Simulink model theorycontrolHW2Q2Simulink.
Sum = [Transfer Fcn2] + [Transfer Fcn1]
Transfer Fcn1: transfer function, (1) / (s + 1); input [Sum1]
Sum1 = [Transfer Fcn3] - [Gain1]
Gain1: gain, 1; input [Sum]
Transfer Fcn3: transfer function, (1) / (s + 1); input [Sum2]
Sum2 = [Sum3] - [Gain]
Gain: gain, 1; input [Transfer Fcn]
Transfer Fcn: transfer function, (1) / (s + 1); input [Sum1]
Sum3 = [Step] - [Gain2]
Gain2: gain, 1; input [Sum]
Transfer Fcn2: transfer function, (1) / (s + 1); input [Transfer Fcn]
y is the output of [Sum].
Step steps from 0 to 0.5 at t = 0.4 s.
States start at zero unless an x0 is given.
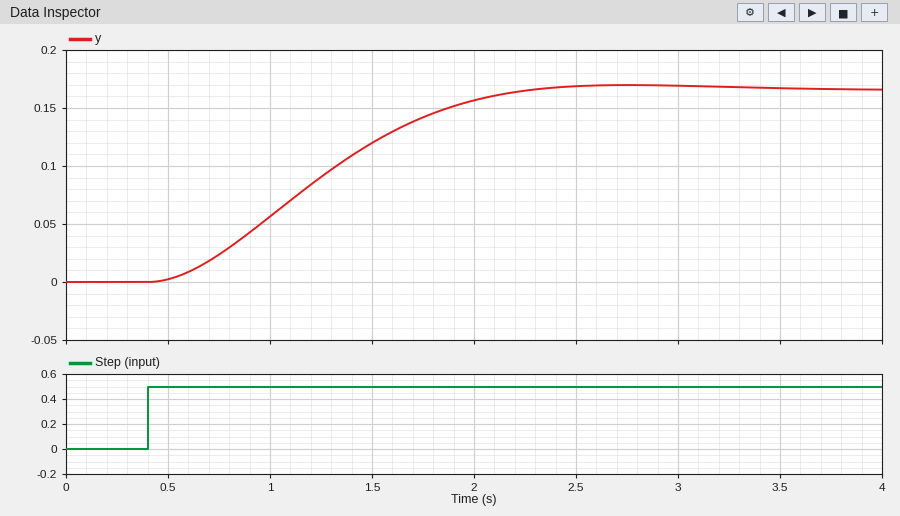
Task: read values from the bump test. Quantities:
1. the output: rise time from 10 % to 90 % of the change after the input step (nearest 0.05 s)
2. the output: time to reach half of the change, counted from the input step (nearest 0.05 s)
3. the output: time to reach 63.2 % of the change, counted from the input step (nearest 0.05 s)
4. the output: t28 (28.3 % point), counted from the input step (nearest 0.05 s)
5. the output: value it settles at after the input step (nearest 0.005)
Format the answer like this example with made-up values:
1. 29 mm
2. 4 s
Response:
1. 1.20 s
2. 0.80 s
3. 0.95 s
4. 0.55 s
5. 0.165
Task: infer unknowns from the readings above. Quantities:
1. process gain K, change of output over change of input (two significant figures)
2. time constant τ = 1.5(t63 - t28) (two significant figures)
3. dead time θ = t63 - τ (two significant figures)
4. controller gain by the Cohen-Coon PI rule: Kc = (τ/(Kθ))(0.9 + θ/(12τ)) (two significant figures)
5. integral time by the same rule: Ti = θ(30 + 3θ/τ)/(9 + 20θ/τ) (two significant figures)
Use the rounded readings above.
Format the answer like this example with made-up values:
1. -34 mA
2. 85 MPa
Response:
1. 0.33
2. 0.60 s
3. 0.35 s
4. 4.9
5. 0.54 s
